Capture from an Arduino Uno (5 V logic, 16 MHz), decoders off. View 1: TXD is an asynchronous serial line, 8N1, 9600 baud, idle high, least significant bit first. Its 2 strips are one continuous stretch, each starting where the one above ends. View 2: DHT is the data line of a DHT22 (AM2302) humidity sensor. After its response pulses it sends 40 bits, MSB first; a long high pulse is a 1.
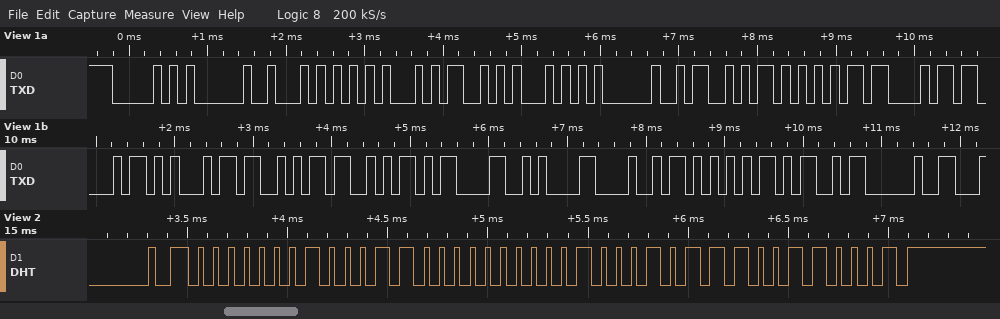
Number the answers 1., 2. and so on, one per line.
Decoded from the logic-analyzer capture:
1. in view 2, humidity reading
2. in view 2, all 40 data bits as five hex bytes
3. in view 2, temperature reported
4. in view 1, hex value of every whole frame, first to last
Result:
1. 28.0 %
2. 01 18 01 17 31
3. 27.9 °C
4. 50 20 54 45 53 54 20 53 55 43 43 45 53 53 0D 0A 48 55 4D 20
